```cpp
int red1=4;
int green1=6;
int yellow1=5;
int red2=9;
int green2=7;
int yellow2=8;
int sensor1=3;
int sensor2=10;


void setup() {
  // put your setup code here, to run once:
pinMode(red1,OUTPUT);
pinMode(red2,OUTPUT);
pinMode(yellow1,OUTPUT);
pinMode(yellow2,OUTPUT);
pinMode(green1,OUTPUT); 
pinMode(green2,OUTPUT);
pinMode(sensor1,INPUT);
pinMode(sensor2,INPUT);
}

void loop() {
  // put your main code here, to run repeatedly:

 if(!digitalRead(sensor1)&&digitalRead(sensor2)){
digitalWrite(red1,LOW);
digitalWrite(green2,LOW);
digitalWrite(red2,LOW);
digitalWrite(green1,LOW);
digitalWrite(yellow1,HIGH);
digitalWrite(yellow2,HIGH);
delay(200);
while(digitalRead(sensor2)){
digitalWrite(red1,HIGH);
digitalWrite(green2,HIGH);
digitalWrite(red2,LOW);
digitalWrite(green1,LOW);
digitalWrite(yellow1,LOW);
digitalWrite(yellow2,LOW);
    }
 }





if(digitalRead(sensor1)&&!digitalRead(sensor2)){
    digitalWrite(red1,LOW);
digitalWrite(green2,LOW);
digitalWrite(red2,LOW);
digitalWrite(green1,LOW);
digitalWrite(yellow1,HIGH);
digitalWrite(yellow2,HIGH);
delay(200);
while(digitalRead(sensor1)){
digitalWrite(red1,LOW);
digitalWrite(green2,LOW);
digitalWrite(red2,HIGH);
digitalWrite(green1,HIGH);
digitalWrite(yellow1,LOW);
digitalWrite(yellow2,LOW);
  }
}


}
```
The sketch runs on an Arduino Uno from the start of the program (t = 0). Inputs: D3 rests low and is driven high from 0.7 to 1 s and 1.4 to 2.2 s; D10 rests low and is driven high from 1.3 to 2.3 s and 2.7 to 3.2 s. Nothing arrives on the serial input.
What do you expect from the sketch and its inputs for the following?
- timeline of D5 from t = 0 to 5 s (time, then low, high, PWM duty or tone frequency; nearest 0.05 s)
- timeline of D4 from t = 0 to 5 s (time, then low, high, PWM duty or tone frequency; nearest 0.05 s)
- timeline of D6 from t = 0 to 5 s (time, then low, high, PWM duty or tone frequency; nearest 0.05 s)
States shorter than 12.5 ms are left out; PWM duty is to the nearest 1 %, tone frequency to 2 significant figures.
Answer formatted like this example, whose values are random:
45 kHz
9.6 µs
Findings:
0 s low; 0.7 s high; 0.9 s low; 1.3 s high; 1.5 s low; 2.7 s high; 2.9 s low
0 s low; 1.5 s high; 2.7 s low; 2.9 s high
0 s low; 0.9 s high; 1.3 s low
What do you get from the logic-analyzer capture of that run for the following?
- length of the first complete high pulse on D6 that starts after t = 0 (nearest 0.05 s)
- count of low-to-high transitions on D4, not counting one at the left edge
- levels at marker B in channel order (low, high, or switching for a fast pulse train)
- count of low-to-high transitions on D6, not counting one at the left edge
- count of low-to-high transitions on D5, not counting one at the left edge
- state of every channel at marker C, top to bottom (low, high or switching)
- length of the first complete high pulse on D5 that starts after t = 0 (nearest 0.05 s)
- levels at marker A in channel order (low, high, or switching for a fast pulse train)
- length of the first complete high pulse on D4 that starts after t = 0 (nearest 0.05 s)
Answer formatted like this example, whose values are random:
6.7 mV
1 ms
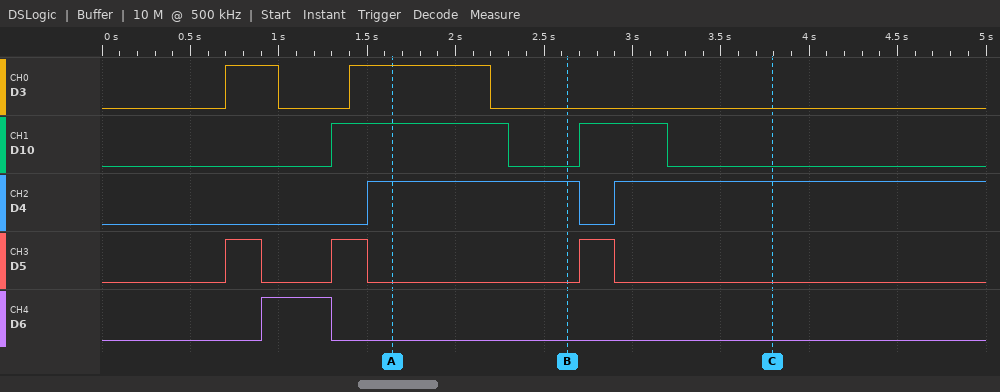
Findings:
0.40 s
2
D3 low, D10 low, D4 high, D5 low, D6 low
1
3
D3 low, D10 low, D4 high, D5 low, D6 low
0.20 s
D3 high, D10 high, D4 high, D5 low, D6 low
1.20 s
